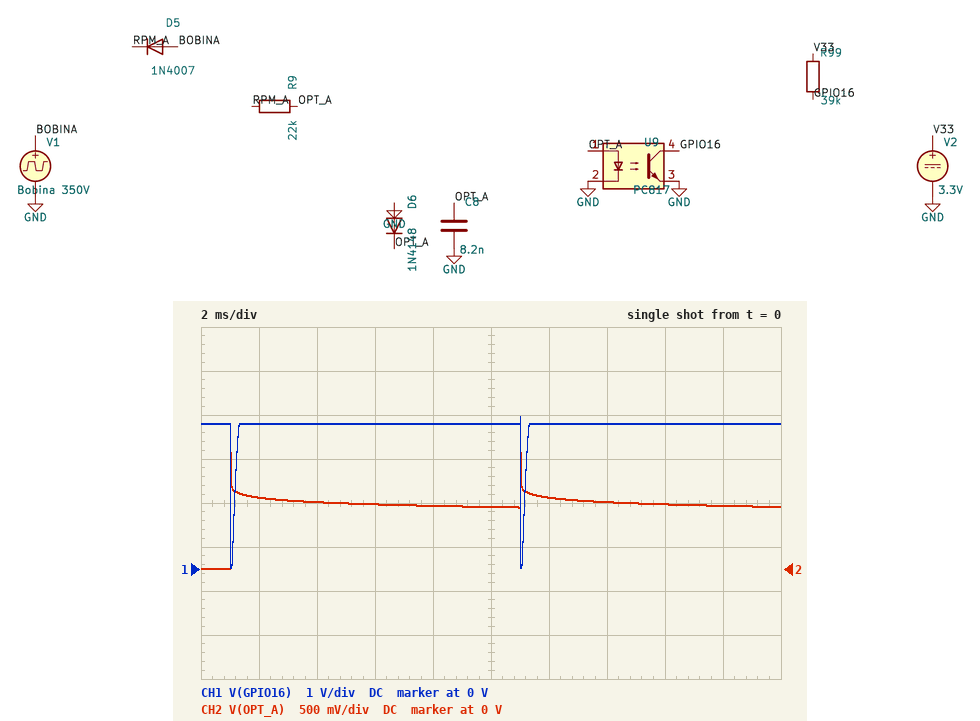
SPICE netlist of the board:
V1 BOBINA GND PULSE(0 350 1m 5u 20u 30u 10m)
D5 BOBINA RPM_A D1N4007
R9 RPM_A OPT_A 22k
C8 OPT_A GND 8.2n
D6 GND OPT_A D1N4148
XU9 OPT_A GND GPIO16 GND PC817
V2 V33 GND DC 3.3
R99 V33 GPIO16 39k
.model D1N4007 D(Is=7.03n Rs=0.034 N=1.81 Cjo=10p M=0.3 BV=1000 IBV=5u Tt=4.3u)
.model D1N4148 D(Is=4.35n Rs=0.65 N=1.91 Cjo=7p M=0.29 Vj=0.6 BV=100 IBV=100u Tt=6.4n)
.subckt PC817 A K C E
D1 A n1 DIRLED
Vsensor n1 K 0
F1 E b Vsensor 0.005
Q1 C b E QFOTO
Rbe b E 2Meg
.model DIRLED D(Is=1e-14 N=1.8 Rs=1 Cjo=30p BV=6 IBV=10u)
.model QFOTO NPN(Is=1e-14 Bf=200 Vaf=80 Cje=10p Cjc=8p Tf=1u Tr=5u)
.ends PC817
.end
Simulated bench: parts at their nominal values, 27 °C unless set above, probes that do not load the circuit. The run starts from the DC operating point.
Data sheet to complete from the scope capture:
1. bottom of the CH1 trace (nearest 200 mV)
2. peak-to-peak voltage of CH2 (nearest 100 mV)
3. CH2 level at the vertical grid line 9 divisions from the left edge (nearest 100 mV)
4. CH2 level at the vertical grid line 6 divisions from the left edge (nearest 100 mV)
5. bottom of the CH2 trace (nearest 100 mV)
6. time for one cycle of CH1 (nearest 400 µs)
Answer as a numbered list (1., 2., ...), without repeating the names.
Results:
1. 0 V
2. 1.3 V
3. 700 mV
4. 800 mV
5. 0 V
6. 10.0 ms
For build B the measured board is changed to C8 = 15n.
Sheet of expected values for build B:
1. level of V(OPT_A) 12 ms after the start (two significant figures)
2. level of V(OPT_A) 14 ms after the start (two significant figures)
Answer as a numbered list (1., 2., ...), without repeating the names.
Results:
1. 840 mV
2. 790 mV
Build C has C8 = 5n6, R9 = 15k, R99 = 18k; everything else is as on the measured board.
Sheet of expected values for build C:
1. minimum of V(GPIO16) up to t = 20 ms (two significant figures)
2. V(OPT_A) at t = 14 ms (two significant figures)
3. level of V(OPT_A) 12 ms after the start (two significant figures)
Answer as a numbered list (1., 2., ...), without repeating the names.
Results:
1. 33 mV
2. 720 mV
3. 750 mV
